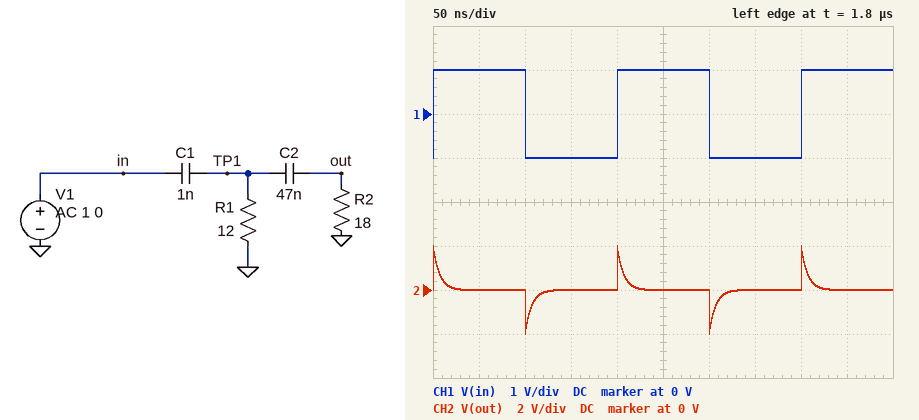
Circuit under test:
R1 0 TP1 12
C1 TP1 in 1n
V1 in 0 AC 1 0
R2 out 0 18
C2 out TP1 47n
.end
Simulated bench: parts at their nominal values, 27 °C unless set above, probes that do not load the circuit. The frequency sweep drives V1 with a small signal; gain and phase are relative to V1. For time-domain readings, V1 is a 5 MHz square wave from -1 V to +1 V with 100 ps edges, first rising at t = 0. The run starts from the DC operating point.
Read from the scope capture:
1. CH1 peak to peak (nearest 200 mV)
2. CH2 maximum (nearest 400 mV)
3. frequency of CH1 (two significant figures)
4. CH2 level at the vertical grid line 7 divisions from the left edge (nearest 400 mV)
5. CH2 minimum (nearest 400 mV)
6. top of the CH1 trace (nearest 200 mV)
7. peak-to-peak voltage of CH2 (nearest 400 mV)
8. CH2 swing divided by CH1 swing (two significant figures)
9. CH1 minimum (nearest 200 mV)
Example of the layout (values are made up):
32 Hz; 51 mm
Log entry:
2.0 V; 2.0 V; 5.0 MHz; 0 V; -2.0 V; 1.0 V; 4.0 V; 2.0; -1.0 V
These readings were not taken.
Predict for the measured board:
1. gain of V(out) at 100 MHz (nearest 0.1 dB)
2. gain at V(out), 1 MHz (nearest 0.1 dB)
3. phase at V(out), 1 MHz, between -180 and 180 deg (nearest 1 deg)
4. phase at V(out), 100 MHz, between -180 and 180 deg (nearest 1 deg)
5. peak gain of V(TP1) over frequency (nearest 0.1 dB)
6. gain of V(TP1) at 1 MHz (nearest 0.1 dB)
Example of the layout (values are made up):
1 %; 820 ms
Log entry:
-0.2 dB; -27.0 dB; 94 deg; 13 deg; 0 dB; -26.8 dB
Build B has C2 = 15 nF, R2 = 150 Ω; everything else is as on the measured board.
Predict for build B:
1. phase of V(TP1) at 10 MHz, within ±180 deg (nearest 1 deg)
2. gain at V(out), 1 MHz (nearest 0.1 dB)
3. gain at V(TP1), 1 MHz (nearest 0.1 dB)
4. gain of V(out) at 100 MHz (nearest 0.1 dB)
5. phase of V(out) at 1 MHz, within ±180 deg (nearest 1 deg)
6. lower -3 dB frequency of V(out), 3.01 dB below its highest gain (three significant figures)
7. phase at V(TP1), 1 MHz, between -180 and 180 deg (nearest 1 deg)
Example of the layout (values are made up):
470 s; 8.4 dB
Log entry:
55 deg; -23.2 dB; -23.1 dB; -0.1 dB; 90 deg; 14.3 MHz; 86 deg
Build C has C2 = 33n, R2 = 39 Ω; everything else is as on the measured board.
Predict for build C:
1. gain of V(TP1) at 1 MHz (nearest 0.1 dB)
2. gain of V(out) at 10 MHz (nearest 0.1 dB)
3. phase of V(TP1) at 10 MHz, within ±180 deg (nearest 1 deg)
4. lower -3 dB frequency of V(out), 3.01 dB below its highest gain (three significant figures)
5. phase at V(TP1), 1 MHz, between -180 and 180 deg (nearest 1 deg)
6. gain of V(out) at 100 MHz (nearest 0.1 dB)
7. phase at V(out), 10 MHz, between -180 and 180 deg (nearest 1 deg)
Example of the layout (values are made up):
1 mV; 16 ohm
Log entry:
-24.8 dB; -6.0 dB; 60 deg; 17.4 MHz; 85 deg; -0.1 dB; 61 deg
